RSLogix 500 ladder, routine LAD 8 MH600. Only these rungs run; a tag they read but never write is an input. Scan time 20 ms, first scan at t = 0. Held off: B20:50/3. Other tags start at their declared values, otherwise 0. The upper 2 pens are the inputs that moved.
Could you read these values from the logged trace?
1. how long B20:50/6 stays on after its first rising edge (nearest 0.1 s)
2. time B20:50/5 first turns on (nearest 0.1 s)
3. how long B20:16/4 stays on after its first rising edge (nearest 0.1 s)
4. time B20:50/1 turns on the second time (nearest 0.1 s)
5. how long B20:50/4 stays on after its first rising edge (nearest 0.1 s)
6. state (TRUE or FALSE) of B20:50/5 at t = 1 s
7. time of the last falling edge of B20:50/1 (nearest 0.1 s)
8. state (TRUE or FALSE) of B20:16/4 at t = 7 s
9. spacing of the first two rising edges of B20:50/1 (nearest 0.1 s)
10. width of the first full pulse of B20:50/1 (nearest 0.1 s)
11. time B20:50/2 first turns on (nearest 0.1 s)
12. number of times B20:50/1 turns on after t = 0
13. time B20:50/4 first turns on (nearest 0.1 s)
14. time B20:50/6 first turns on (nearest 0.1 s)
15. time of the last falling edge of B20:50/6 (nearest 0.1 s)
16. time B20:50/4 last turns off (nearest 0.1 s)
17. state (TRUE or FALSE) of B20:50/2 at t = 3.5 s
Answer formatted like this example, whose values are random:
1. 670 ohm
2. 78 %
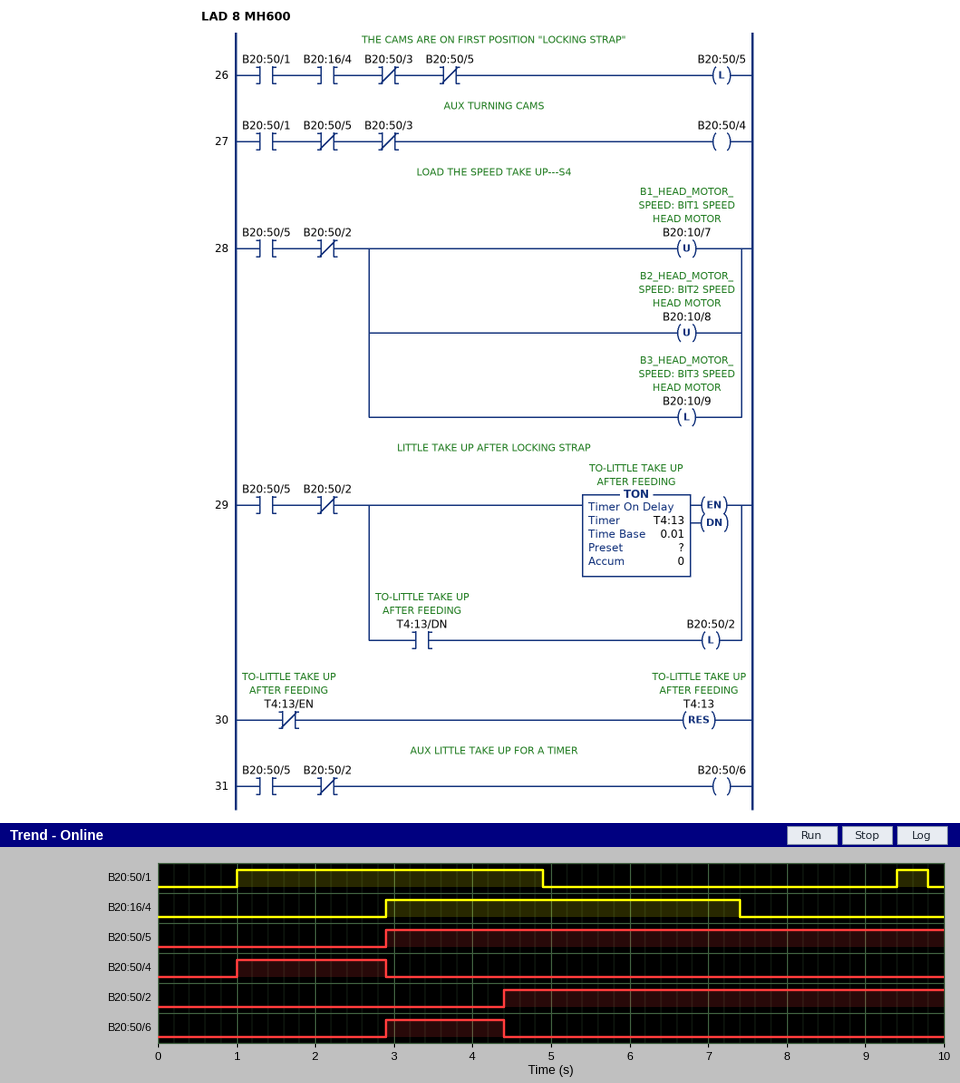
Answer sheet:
1. 1.5 s
2. 2.9 s
3. 4.5 s
4. 9.4 s
5. 1.9 s
6. FALSE
7. 9.8 s
8. TRUE
9. 8.4 s
10. 3.9 s
11. 4.4 s
12. 2
13. 1.0 s
14. 2.9 s
15. 4.4 s
16. 2.9 s
17. FALSE
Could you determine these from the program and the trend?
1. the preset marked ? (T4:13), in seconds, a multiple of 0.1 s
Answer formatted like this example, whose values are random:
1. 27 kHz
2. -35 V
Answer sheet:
1. 1.5 s
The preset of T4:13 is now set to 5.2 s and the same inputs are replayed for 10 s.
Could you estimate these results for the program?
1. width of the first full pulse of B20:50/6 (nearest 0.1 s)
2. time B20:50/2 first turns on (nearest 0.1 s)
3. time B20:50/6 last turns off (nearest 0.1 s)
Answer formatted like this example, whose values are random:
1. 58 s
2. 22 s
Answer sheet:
1. 5.2 s
2. 8.1 s
3. 8.1 s
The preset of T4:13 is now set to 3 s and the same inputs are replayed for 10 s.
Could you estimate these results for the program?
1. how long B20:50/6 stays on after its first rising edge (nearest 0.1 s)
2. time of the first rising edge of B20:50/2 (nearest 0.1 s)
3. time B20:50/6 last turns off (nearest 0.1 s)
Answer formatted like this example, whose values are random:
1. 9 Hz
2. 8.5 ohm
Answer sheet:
1. 3.0 s
2. 5.9 s
3. 5.9 s
